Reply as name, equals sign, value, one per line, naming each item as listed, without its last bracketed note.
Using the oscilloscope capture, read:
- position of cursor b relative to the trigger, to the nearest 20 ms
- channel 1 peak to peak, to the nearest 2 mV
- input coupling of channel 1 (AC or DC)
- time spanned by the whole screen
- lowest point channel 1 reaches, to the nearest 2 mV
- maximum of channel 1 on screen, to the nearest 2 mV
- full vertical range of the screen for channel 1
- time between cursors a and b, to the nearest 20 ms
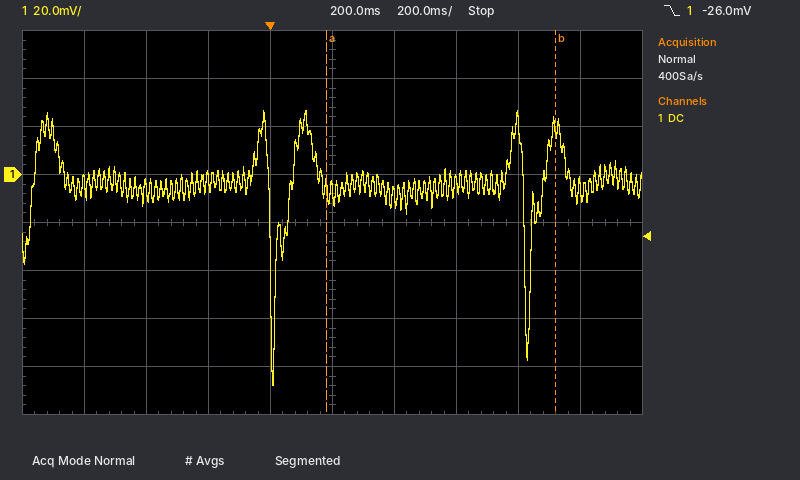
position of cursor b relative to the trigger, to the nearest 20 ms = +920 ms
channel 1 peak to peak, to the nearest 2 mV = 114 mV
input coupling of channel 1 = DC
time spanned by the whole screen = 2 s
lowest point channel 1 reaches, to the nearest 2 mV = -88 mV
maximum of channel 1 on screen, to the nearest 2 mV = 26 mV
full vertical range of the screen for channel 1 = 160 mV
time between cursors a and b, to the nearest 20 ms = 740 ms
